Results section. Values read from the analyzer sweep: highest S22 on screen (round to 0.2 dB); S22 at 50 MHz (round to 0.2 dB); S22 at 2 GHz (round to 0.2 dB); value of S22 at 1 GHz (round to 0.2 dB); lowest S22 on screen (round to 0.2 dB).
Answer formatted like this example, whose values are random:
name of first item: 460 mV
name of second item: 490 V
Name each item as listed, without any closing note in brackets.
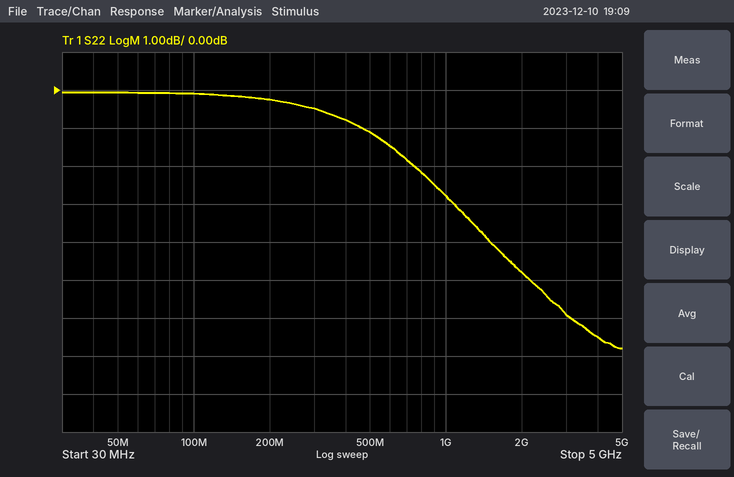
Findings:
highest S22 on screen: 0.0 dB
S22 at 50 MHz: 0.0 dB
S22 at 2 GHz: -4.8 dB
value of S22 at 1 GHz: -2.8 dB
lowest S22 on screen: -6.8 dB
